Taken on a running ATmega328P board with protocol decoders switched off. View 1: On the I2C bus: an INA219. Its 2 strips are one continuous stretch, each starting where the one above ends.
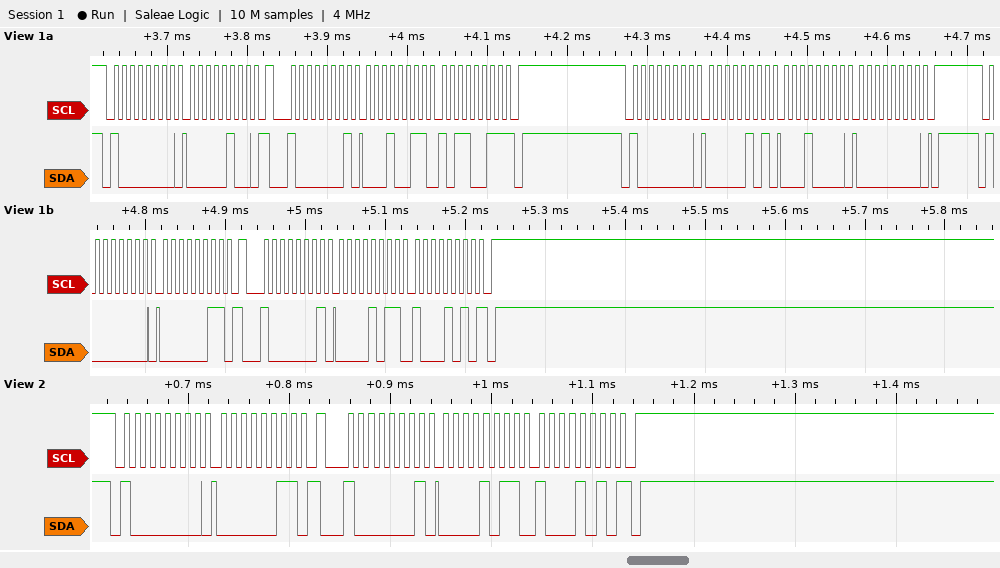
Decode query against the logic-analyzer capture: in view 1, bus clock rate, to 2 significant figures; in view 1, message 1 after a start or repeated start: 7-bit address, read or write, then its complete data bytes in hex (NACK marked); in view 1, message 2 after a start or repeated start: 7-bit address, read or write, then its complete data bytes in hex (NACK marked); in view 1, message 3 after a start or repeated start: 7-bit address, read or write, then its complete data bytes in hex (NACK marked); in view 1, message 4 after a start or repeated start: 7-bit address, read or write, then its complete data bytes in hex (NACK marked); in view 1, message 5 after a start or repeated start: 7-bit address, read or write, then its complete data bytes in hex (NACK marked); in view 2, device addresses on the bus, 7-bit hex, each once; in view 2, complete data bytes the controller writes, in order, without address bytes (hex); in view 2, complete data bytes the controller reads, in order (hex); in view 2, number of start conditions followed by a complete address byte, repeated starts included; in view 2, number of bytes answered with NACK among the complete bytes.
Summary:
100 kHz
0x40 write: 04
0x40 read: 13 B3 NACK
0x40 write: 05 10 00
0x40 write: 03
0x40 read: 0B 8A NACK
0x40
03
0B 8A
2
1
